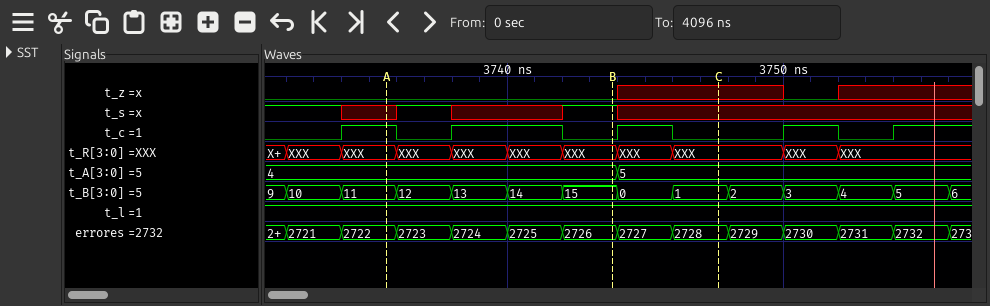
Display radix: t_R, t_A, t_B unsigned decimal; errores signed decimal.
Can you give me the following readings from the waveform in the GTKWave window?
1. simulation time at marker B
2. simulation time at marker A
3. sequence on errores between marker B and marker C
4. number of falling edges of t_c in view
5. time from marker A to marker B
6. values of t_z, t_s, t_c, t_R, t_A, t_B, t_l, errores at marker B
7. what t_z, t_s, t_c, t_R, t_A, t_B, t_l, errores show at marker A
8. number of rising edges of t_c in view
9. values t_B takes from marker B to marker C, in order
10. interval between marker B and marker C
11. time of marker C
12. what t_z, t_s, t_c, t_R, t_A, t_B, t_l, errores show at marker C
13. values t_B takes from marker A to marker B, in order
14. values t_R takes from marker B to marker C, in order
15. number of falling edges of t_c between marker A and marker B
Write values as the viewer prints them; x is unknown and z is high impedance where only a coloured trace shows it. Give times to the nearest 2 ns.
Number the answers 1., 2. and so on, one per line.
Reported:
1. 3744 ns
2. 3736 ns
3. 2726, 2727, 2728
4. 4
5. 8 ns
6. t_z=0, t_s=1, t_c=0, t_R=XXX, t_A=4, t_B=15, t_l=1, errores=2726
7. t_z=0, t_s=x, t_c=1, t_R=XXX, t_A=4, t_B=11, t_l=1, errores=2722
8. 5
9. 15, 0, 1
10. 4 ns
11. 3748 ns
12. t_z=x, t_s=x, t_c=0, t_R=XXX, t_A=5, t_B=1, t_l=1, errores=2728
13. 11, 12, 13, 14, 15
14. XXX, XXX, XXX
15. 2
